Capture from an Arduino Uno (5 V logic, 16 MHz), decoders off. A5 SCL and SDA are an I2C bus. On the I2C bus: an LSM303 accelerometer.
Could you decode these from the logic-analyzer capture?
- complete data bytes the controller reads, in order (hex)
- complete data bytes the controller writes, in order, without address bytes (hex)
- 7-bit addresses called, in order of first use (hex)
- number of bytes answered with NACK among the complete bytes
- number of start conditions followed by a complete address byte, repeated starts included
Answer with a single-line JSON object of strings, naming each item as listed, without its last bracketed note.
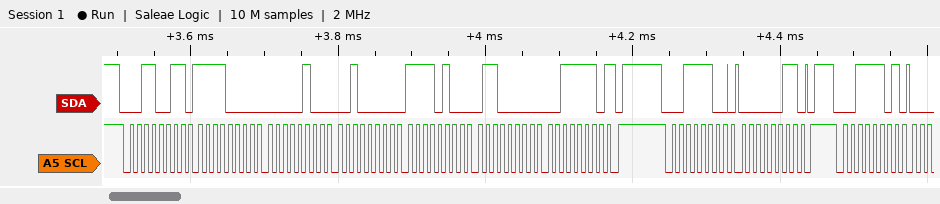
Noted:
{"complete data bytes the controller reads, in order": "F0 04 20 F4 60 3E", "complete data bytes the controller writes, in order, without address bytes": "03", "7-bit addresses called, in order of first use": "0x19 0x1E", "number of bytes answered with NACK among the complete bytes": "1", "number of start conditions followed by a complete address byte, repeated starts included": "3"}
